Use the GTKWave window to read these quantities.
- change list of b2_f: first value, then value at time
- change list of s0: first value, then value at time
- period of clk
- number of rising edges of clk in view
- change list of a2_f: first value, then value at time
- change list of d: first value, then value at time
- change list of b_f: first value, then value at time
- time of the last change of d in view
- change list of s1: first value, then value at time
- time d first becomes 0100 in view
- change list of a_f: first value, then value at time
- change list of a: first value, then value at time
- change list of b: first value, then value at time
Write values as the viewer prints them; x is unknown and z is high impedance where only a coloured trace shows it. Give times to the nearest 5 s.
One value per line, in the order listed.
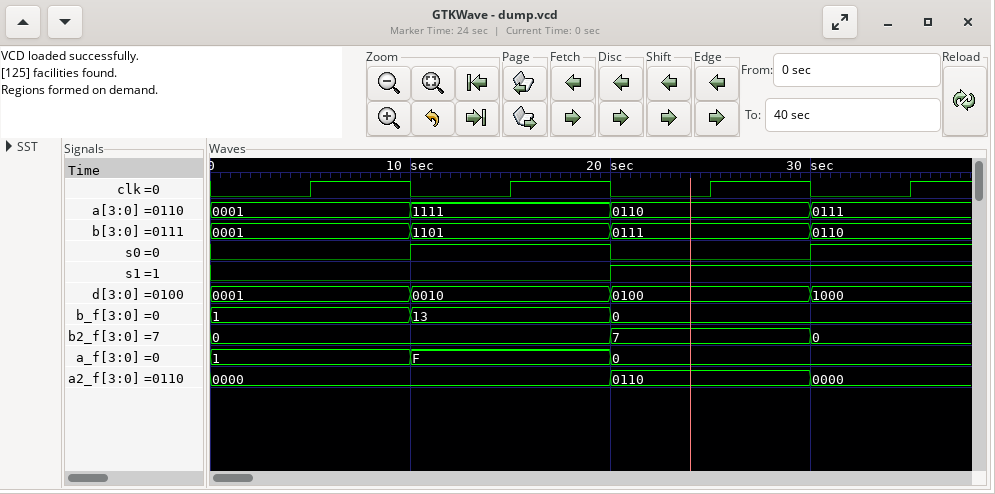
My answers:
0, 7 at 20 s, 0 at 30 s
0, 1 at 10 s, 0 at 20 s, 1 at 30 s
10 s
4
0000, 0110 at 20 s, 0000 at 30 s
0001, 0010 at 10 s, 0100 at 20 s, 1000 at 30 s
1, 13 at 10 s, 0 at 20 s
30 s
0, 1 at 20 s
20 s
1, F at 10 s, 0 at 20 s
0001, 1111 at 10 s, 0110 at 20 s, 0111 at 30 s
0001, 1101 at 10 s, 0111 at 20 s, 0110 at 30 s
